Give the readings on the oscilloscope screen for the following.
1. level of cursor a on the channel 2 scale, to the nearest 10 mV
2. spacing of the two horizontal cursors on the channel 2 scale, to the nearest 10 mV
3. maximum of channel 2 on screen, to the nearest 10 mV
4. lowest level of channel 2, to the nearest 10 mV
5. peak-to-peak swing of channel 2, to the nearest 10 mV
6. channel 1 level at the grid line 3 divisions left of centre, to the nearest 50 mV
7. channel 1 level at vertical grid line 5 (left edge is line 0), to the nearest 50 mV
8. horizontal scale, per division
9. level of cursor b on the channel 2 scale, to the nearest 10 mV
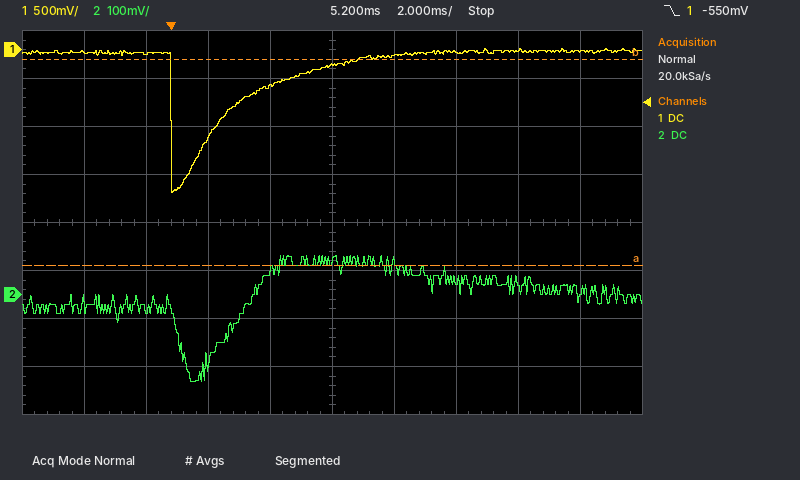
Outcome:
60 mV
430 mV
80 mV
-180 mV
260 mV
-50 mV
-150 mV
2 ms
490 mV
